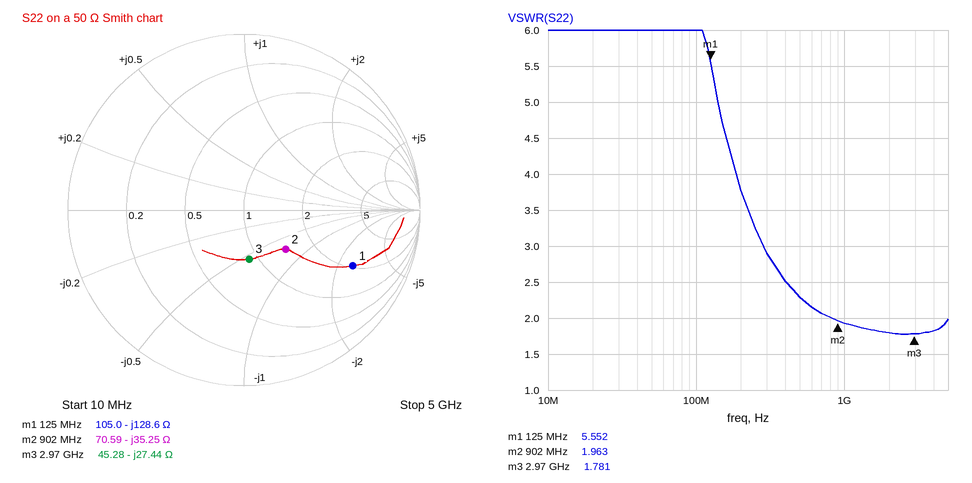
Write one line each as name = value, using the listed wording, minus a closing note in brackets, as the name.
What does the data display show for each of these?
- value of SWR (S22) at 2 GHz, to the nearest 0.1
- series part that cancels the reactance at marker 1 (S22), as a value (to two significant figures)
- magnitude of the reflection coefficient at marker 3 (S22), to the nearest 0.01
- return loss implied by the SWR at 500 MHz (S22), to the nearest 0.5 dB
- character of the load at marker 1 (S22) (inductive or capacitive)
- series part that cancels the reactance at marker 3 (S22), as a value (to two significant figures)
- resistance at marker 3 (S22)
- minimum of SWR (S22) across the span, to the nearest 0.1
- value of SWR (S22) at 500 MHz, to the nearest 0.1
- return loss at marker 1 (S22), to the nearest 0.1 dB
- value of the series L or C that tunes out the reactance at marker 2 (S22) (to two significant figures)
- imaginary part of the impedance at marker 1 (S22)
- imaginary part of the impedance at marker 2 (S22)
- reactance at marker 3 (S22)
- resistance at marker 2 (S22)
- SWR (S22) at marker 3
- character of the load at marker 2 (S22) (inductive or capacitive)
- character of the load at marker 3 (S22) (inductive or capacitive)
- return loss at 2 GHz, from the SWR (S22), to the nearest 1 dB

value of SWR (S22) at 2 GHz, to the nearest 0.1 = 1.8
series part that cancels the reactance at marker 1 (S22), as a value = 160 nH
magnitude of the reflection coefficient at marker 3 (S22), to the nearest 0.01 = 0.28
return loss implied by the SWR at 500 MHz (S22), to the nearest 0.5 dB = 8.0 dB
character of the load at marker 1 (S22) = capacitive
series part that cancels the reactance at marker 3 (S22), as a value = 1.5 nH
resistance at marker 3 = 45.28 Ω
minimum of SWR (S22) across the span, to the nearest 0.1 = 1.8
value of SWR (S22) at 500 MHz, to the nearest 0.1 = 2.3
return loss at marker 1 (S22), to the nearest 0.1 dB = 3.2 dB
value of the series L or C that tunes out the reactance at marker 2 (S22) = 6.2 nH
imaginary part of the impedance at marker 1 = -128.6 Ω
imaginary part of the impedance at marker 2 = -35.25 Ω
reactance at marker 3 = -27.44 Ω
resistance at marker 2 = 70.59 Ω
SWR (S22) at marker 3 = 1.781
character of the load at marker 2 (S22) = capacitive
character of the load at marker 3 (S22) = capacitive
return loss at 2 GHz, from the SWR (S22), to the nearest 1 dB = 11 dB
